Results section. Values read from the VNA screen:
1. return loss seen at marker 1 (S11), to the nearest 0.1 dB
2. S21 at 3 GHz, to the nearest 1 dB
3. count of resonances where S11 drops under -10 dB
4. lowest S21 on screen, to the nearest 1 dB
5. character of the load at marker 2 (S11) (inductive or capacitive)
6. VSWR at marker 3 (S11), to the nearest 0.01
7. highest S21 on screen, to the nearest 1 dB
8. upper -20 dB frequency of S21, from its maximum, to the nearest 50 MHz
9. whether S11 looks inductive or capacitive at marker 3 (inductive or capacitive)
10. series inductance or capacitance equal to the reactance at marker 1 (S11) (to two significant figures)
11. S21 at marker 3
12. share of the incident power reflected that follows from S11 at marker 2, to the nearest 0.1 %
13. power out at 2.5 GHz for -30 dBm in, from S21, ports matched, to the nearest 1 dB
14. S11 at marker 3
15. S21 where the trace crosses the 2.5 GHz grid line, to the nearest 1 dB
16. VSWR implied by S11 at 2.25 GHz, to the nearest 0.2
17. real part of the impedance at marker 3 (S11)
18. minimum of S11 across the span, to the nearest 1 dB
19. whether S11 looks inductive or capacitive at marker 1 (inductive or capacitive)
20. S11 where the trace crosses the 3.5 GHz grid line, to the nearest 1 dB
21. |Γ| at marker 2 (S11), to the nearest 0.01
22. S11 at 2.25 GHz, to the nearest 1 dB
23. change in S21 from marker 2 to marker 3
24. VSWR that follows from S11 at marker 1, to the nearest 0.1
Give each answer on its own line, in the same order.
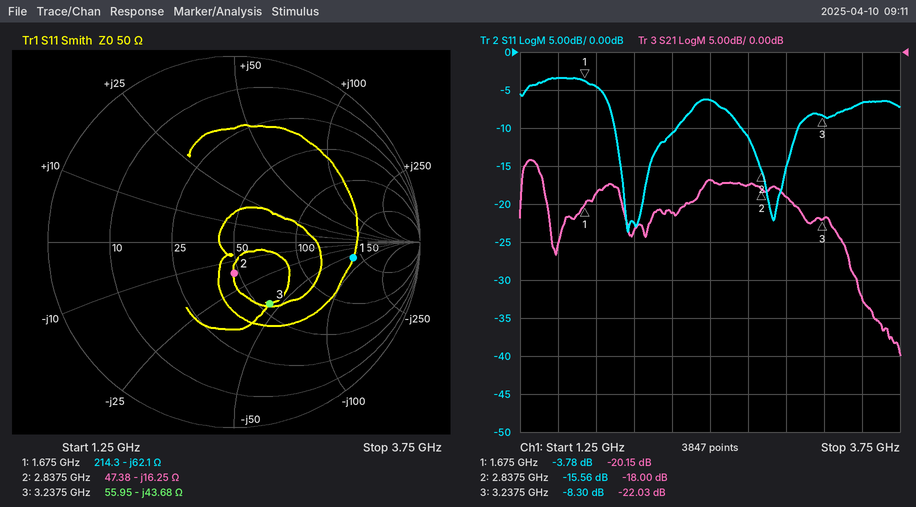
3.8 dB
-19 dB
2
-40 dB
capacitive
2.25
-14 dB
3.55 GHz
capacitive
1.5 pF
-22.03 dB
2.8 %
-47 dBm
-8.30 dB
-17 dB
1.8
55.95 Ω
-24 dB
capacitive
-7 dB
0.17
-11 dB
-4.03 dB
4.7
